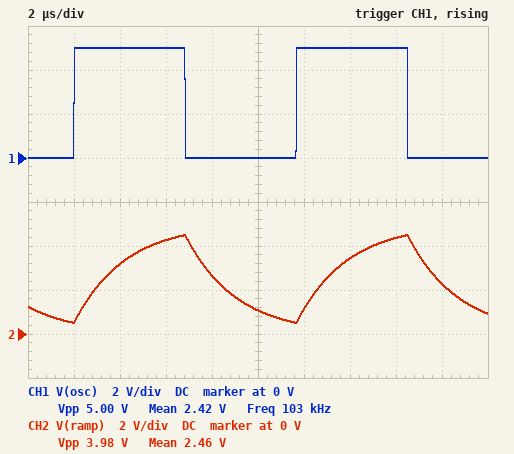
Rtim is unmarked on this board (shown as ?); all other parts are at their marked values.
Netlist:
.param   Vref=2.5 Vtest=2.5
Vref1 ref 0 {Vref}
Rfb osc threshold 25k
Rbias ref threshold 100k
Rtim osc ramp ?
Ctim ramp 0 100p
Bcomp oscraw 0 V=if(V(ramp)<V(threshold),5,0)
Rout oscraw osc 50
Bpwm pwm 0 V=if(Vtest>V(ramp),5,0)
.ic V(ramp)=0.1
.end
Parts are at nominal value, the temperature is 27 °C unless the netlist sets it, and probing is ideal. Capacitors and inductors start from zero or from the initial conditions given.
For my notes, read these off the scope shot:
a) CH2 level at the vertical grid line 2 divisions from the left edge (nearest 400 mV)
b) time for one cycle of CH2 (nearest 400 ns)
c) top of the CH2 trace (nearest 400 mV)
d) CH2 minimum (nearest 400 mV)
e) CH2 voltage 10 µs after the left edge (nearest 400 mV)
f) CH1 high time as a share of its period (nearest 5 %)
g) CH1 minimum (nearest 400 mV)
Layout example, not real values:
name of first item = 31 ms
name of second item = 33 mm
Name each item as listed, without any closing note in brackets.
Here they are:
CH2 level at the vertical grid line 2 divisions from the left edge = 3.2 V
time for one cycle of CH2 = 9.6 µs
top of the CH2 trace = 4.4 V
CH2 minimum = 400 mV
CH2 voltage 10 µs after the left edge = 1.2 V
CH1 high time as a share of its period = 50 %
CH1 minimum = 0 V
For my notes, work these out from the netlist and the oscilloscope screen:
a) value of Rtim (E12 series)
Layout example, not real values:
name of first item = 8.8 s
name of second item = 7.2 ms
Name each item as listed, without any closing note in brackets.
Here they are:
value of Rtim = 22 kΩ
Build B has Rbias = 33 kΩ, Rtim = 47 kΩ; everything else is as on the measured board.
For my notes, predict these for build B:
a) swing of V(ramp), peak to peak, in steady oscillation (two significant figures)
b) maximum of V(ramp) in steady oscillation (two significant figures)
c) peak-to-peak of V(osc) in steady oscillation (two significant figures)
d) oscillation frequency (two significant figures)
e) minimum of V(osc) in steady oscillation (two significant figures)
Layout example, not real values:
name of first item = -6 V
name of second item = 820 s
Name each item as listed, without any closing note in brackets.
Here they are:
swing of V(ramp), peak to peak, in steady oscillation = 2.8 V
maximum of V(ramp) in steady oscillation = 3.9 V
peak-to-peak of V(osc) in steady oscillation = 5.0 V
oscillation frequency = 82 kHz
minimum of V(osc) in steady oscillation = 3.3 mV
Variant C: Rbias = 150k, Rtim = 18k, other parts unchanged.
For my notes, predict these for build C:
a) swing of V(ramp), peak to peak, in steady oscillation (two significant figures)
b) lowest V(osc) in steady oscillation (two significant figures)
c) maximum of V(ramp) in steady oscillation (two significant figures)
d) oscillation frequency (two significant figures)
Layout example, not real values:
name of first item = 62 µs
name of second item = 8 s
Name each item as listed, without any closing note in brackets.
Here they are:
swing of V(ramp), peak to peak, in steady oscillation = 4.3 V
lowest V(osc) in steady oscillation = 1.7 mV
maximum of V(ramp) in steady oscillation = 4.6 V
oscillation frequency = 110 kHz
